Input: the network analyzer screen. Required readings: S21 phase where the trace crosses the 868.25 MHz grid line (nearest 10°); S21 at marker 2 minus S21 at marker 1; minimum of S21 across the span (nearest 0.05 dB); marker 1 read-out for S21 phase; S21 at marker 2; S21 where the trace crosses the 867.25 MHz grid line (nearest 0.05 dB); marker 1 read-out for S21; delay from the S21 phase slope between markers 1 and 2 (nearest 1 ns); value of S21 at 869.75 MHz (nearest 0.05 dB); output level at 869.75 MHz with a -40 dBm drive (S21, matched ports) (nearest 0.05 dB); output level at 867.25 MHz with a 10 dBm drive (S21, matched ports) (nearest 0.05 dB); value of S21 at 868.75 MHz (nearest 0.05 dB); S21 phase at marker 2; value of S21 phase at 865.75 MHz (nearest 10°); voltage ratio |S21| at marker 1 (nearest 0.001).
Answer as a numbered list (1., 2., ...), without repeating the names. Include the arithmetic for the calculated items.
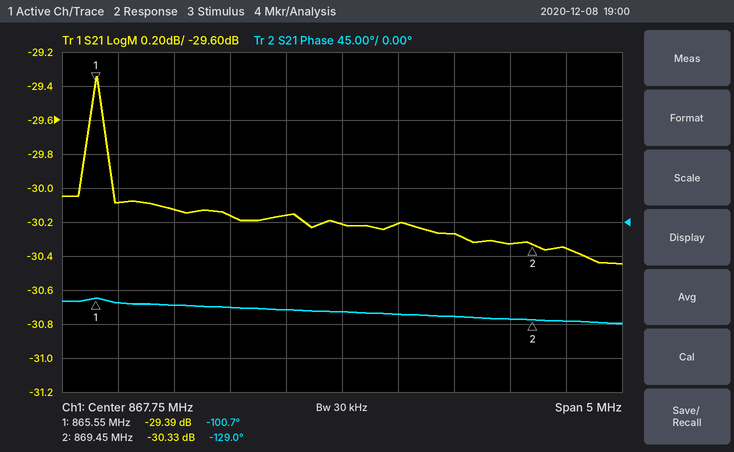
1. -120°
2. -30.33 − (-29.39) = -0.94 dB
3. -30.45 dB
4. -100.7°
5. -30.33 dB
6. -30.15 dB
7. -29.39 dB
8. −(-129° − (-100.7°))/(360° × 3.9 MHz) ≈ 20 ns
9. -30.35 dB
10. -40 dBm + (-30.35 dB) = -70.35 dBm
11. 10 dBm + (-30.15 dB) = -20.15 dBm
12. -30.25 dB
13. -129.0°
14. -110°
15. 10^(-29.39/20) ≈ 0.034
